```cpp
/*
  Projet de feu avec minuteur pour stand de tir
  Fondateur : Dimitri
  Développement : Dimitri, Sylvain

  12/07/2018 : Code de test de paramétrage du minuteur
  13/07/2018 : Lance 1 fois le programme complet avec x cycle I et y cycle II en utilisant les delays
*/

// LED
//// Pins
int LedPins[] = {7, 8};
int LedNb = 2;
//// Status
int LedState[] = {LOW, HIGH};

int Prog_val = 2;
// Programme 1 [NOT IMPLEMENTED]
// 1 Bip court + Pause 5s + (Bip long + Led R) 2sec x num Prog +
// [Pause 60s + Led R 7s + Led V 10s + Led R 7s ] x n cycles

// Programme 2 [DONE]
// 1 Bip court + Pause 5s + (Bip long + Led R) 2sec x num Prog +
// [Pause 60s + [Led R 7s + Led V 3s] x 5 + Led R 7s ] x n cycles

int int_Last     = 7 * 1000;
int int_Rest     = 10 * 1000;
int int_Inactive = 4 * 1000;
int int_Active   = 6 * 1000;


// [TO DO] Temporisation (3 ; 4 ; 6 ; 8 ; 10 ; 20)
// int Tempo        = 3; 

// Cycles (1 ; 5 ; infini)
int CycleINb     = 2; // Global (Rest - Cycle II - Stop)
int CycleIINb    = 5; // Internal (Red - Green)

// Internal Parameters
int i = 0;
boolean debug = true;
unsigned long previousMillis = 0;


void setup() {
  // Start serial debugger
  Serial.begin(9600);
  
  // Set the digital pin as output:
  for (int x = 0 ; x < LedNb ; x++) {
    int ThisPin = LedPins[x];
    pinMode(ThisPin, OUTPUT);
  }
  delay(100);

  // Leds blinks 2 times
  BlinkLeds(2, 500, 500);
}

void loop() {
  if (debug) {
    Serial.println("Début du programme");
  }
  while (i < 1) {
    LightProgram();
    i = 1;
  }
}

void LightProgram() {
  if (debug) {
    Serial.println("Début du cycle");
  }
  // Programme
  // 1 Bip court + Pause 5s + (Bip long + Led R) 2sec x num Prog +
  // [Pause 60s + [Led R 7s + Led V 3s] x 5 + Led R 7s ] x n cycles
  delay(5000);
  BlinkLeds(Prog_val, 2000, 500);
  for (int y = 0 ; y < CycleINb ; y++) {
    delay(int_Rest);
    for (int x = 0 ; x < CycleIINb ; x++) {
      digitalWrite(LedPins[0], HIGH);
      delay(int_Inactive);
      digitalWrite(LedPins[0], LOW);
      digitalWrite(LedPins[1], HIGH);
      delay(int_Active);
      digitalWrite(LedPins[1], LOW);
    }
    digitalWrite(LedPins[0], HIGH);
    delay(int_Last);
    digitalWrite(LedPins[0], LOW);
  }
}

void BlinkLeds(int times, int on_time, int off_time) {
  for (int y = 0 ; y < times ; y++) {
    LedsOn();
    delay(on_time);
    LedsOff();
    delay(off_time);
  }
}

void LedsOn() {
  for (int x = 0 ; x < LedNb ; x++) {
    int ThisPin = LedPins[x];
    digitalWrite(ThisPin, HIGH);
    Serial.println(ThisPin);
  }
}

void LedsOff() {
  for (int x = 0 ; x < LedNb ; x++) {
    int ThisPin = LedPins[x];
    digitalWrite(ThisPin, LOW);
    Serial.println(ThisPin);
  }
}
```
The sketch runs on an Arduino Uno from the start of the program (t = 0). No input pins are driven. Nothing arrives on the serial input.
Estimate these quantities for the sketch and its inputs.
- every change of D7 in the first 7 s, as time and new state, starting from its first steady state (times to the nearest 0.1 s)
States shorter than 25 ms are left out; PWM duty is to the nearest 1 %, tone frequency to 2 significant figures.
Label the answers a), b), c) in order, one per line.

a) 0 s low; 0.1 s high; 0.6 s low; 1.1 s high; 1.6 s low
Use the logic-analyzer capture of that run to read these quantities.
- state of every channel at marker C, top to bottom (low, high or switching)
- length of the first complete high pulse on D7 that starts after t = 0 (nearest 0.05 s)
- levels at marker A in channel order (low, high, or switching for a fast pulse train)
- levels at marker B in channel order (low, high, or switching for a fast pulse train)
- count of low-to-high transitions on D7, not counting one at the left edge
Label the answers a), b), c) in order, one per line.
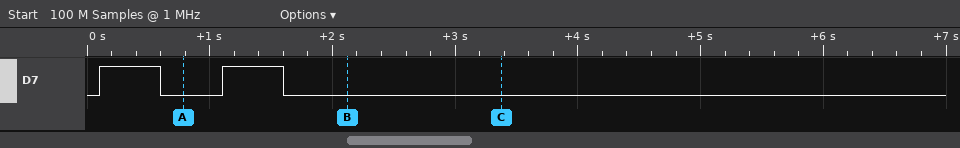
a) D7 low
b) 0.50 s
c) D7 low
d) D7 low
e) 2
